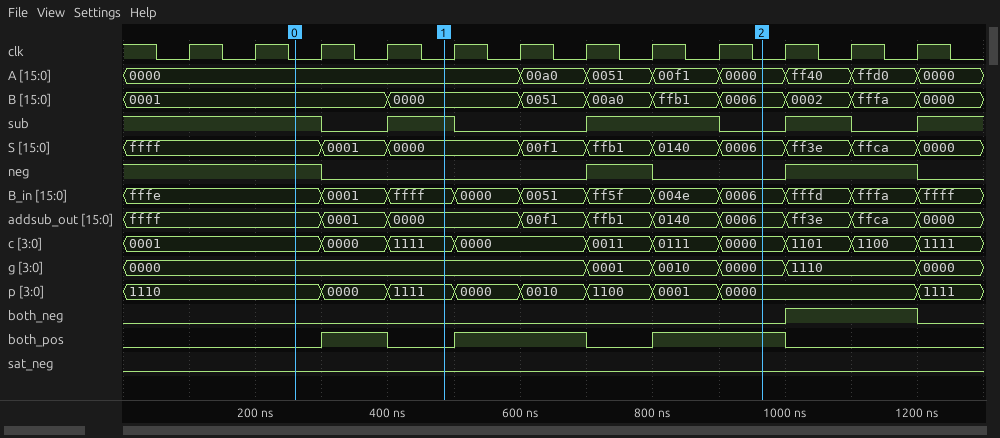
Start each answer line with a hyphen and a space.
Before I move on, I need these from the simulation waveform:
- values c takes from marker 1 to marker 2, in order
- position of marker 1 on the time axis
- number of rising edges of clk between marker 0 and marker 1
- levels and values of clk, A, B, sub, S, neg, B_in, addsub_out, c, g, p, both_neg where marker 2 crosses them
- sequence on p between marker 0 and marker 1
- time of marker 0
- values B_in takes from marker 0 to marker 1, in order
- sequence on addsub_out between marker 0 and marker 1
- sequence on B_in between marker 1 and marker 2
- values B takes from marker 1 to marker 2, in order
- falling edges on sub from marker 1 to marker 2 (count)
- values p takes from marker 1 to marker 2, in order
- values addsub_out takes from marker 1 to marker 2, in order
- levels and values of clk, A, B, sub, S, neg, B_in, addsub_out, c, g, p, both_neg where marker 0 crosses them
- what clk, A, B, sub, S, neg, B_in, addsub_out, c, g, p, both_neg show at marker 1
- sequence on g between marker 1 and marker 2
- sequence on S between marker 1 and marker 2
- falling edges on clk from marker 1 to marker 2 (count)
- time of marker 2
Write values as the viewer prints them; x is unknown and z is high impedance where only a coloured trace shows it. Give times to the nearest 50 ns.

- 1111, 0000, 0011, 0111, 0000
- 500 ns
- 2
- clk=0, A=0000, B=0006, sub=0, S=0006, neg=0, B_in=0006, addsub_out=0006, c=0000, g=0000, p=0000, both_neg=0
- 1110, 0000, 1111
- 250 ns
- fffe, 0001, ffff
- ffff, 0001, 0000
- ffff, 0000, 0051, ff5f, 004e, 0006
- 0000, 0051, 00a0, ffb1, 0006
- 2
- 1111, 0000, 0010, 1100, 0001, 0000
- 0000, 00f1, ffb1, 0140, 0006
- clk=0, A=0000, B=0001, sub=1, S=ffff, neg=1, B_in=fffe, addsub_out=ffff, c=0001, g=0000, p=1110, both_neg=0
- clk=0, A=0000, B=0000, sub=1, S=0000, neg=0, B_in=ffff, addsub_out=0000, c=1111, g=0000, p=1111, both_neg=0
- 0000, 0001, 0010, 0000
- 0000, 00f1, ffb1, 0140, 0006
- 5
- 950 ns
